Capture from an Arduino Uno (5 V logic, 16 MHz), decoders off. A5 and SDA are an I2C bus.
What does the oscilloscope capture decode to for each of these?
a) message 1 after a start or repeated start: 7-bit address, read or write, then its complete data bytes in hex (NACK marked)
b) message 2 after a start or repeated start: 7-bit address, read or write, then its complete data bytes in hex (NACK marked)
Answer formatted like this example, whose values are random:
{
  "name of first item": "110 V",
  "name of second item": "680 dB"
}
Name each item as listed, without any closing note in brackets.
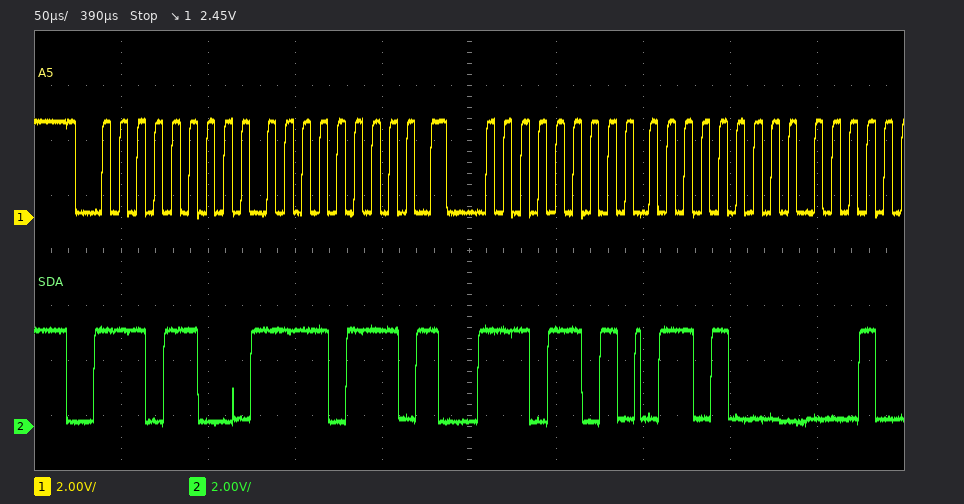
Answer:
{
  "message 1 after a start or repeated start: 7-bit address, read or write, then its complete data bytes in hex": "0x76 write: F7",
  "message 2 after a start or repeated start: 7-bit address, read or write, then its complete data bytes in hex": "0x76 read: 68"
}
